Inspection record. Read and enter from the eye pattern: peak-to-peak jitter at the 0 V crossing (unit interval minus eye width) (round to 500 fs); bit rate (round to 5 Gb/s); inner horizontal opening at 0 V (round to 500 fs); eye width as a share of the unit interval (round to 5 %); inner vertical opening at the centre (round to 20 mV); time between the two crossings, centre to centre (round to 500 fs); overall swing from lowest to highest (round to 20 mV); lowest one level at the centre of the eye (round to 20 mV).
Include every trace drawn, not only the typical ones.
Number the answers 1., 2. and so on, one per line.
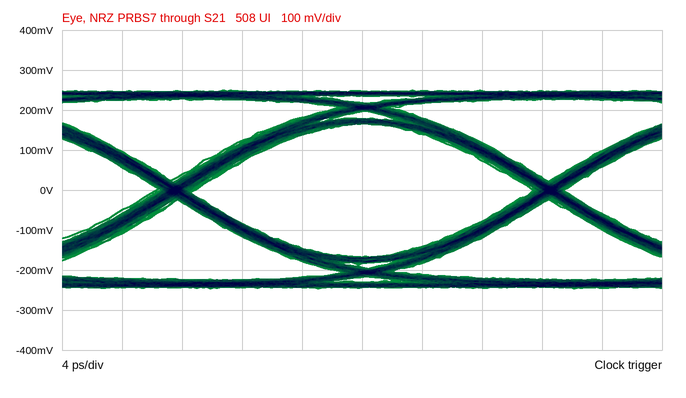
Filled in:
1. 2.5 ps
2. 40 Gb/s
3. 22.5 ps
4. 90 %
5. 340 mV
6. 25.0 ps
7. 500 mV
8. 160 mV
